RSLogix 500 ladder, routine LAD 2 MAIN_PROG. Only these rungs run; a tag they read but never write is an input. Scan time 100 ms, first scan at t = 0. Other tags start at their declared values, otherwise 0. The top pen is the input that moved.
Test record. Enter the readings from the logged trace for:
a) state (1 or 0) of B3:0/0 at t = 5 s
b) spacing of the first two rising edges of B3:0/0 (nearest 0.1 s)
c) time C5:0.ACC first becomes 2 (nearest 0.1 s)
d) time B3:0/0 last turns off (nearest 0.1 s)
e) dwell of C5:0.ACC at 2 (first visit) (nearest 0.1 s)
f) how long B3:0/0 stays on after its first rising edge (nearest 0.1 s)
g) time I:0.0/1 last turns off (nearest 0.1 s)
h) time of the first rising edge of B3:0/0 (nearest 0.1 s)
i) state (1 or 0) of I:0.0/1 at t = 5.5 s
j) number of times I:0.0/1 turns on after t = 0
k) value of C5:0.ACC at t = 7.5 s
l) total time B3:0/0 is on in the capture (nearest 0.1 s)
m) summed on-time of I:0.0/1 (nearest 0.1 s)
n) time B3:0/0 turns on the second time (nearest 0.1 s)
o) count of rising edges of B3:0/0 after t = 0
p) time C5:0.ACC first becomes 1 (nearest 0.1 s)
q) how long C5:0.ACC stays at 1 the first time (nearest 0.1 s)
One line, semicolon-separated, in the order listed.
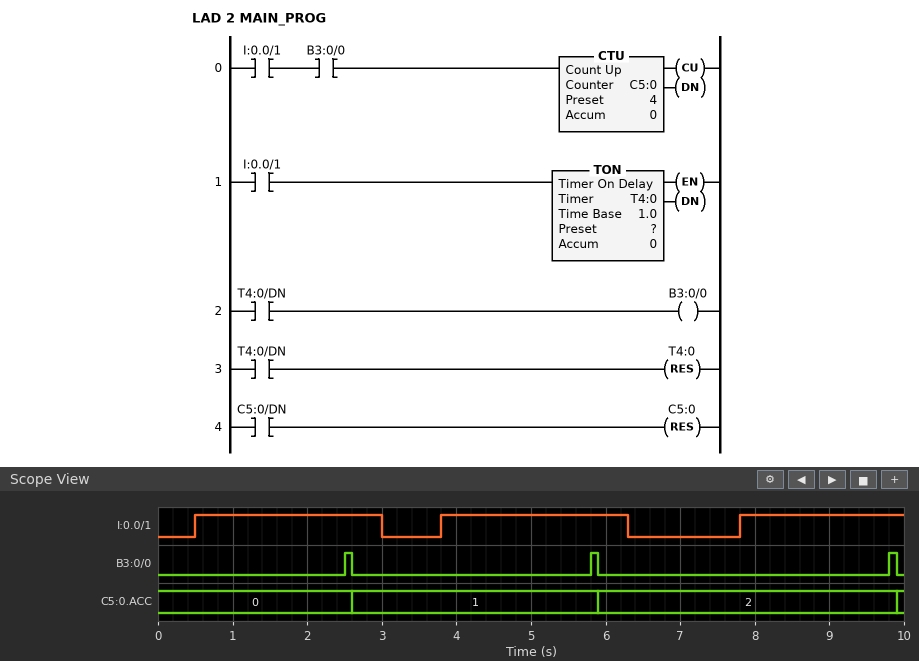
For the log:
0; 3.3 s; 5.9 s; 9.9 s; 4.0 s; 0.1 s; 6.3 s; 2.5 s; 1; 3; 2; 0.3 s; 7.2 s; 5.8 s; 3; 2.6 s; 3.3 s
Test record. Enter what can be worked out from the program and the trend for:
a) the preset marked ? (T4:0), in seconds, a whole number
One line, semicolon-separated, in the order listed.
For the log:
2 s
